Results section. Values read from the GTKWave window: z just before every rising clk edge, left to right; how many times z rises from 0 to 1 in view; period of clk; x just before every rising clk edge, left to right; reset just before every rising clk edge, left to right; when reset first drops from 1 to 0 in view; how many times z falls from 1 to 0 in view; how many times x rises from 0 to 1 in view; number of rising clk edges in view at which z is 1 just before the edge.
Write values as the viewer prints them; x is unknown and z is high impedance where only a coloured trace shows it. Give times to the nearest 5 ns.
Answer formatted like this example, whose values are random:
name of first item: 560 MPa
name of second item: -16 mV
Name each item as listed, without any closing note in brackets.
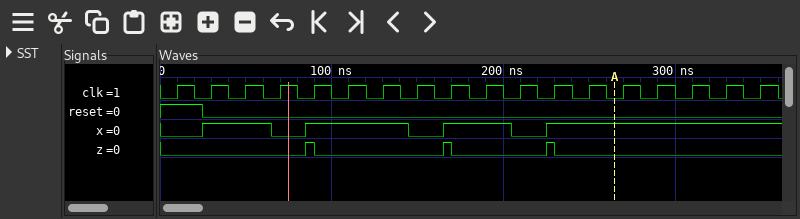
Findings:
z just before every rising clk edge, left to right: 0 0 0 0 1 0 0 0 1 0 0 1 0 0 0 0 0 0
how many times z rises from 0 to 1 in view: 3
period of clk: 20 ns
x just before every rising clk edge, left to right: 0 1 1 0 1 1 1 0 1 1 0 1 1 1 1 1 1 1
reset just before every rising clk edge, left to right: 1 0 0 0 0 0 0 0 0 0 0 0 0 0 0 0 0 0
when reset first drops from 1 to 0 in view: 25 ns
how many times z falls from 1 to 0 in view: 3
how many times x rises from 0 to 1 in view: 4
number of rising clk edges in view at which z is 1 just before the edge: 3
